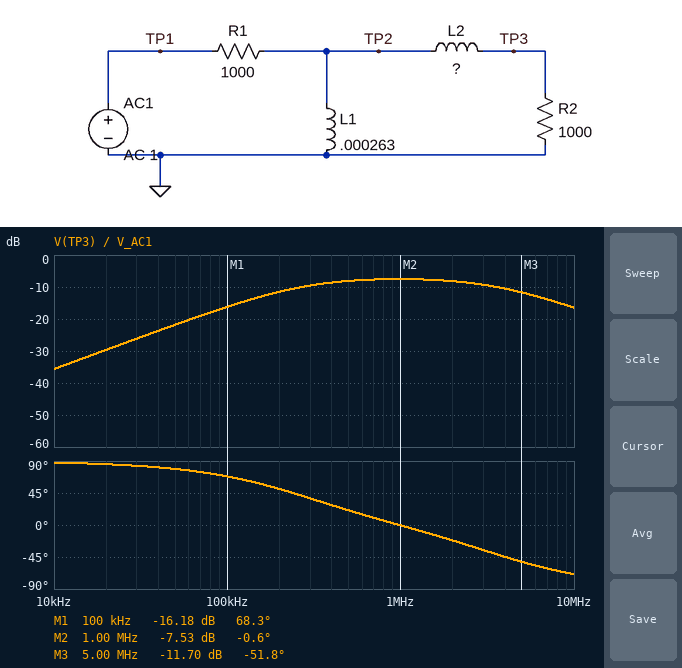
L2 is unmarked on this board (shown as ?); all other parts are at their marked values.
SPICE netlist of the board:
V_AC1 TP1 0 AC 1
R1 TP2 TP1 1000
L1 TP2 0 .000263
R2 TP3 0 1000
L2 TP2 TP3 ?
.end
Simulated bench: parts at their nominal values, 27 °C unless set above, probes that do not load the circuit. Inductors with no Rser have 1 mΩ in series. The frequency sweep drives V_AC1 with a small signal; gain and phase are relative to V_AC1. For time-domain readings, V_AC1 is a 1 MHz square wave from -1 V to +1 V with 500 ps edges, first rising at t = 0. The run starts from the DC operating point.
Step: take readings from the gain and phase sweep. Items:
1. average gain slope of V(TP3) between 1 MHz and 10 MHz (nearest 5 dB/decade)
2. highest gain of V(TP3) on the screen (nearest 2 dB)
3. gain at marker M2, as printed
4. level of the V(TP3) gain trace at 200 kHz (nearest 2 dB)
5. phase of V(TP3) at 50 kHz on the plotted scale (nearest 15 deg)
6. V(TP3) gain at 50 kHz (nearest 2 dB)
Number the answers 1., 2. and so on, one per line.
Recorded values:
1. -10 dB/decade
2. -8 dB
3. -7.53 dB
4. -12 dB
5. 75 deg
6. -22 dB
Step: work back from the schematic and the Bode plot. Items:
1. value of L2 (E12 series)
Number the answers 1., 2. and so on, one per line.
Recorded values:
1. 100 µH
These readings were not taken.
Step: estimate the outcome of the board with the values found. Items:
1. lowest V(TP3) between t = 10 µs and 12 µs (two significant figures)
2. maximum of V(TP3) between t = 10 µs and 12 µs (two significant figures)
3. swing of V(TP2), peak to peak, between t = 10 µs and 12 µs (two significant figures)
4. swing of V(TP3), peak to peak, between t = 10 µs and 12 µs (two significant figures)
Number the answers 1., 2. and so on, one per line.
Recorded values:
1. -500 mV
2. 500 mV
3. 3.5 V
4. 1.0 V
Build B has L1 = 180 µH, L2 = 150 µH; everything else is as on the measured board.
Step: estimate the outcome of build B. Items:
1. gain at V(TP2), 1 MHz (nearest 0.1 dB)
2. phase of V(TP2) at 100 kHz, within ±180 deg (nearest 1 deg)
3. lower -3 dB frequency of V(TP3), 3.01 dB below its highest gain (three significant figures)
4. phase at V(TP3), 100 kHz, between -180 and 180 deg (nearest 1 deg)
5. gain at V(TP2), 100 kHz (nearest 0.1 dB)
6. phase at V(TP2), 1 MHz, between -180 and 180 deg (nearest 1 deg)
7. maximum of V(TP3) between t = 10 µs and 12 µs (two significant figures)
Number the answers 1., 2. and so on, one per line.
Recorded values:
1. -6.3 dB
2. 77 deg
3. 285 kHz
4. 72 deg
5. -19.2 dB
6. 42 deg
7. 420 mV
